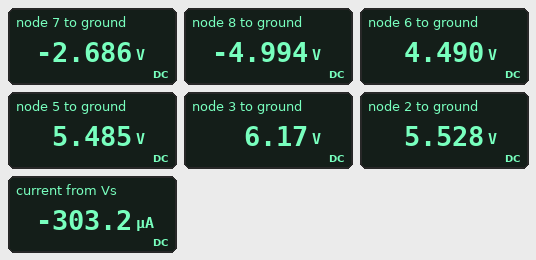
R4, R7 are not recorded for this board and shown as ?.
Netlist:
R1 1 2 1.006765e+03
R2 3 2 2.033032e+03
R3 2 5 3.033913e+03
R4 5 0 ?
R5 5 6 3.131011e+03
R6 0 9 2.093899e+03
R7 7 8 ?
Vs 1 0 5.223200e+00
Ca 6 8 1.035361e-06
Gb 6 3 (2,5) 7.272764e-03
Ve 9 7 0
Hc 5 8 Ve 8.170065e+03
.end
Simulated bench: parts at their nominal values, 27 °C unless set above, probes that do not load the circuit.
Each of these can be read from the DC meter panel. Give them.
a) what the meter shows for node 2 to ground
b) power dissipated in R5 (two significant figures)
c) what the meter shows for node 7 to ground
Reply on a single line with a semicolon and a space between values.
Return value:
5.528 V; 320 µW; -2.686 V
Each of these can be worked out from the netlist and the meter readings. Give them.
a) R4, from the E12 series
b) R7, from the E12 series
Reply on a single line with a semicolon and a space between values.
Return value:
5.6 kΩ; 1.8 kΩ
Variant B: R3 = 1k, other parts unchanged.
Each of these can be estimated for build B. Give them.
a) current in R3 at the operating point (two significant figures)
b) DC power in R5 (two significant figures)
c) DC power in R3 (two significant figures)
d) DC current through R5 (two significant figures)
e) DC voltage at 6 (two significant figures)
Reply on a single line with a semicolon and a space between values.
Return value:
48 µA; 390 µW; 2.3 µW; 350 µA; 4.4 V
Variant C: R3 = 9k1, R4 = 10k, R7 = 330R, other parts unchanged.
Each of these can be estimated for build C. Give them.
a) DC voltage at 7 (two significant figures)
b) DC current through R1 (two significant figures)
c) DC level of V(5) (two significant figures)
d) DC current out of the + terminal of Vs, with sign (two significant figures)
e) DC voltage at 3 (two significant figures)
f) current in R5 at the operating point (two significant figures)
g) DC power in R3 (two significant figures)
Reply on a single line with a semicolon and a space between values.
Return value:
-2.0 V; 410 µA; 5.6 V; -410 µA; 6.5 V; 420 µA; 370 nW
